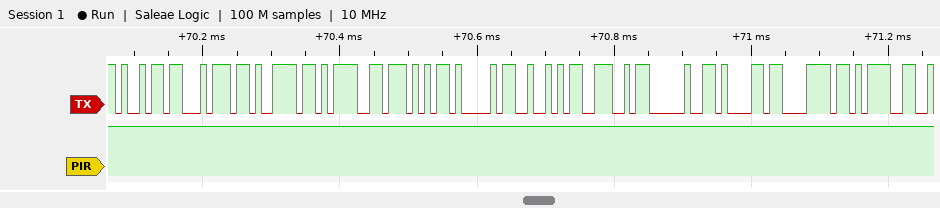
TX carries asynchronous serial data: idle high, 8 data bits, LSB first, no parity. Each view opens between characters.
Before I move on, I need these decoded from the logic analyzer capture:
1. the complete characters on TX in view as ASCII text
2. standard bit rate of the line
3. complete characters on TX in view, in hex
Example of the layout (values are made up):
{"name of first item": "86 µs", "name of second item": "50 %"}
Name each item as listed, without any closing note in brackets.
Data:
{"the complete characters on TX in view as ASCII text": "\"ity=WARN ax=\"", "standard bit rate of the line": "115200 baud", "complete characters on TX in view, in hex": "69, 74, 79, 3D, 57, 41, 52, 4E, 20, 61, 78, 3D"}
